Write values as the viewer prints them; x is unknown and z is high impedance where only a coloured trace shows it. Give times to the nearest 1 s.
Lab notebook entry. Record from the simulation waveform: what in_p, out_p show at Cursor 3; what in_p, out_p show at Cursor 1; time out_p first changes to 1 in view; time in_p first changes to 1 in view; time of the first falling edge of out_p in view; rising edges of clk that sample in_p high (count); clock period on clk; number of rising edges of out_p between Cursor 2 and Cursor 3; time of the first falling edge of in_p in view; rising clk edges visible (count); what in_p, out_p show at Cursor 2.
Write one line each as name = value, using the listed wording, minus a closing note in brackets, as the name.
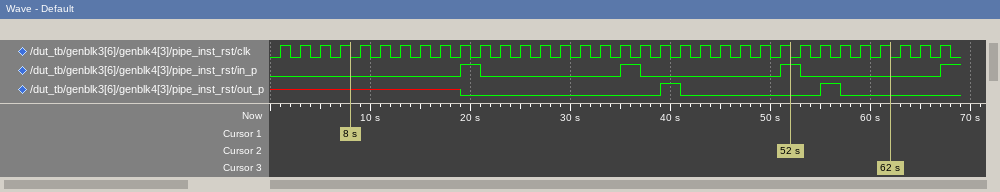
what in_p, out_p show at Cursor 3 = in_p=0, out_p=0
what in_p, out_p show at Cursor 1 = in_p=0, out_p=x
time out_p first changes to 1 in view = 39 s
time in_p first changes to 1 in view = 19 s
time of the first falling edge of out_p in view = 41 s
rising edges of clk that sample in_p high = 3
clock period on clk = 2 s
number of rising edges of out_p between Cursor 2 and Cursor 3 = 1
time of the first falling edge of in_p in view = 21 s
rising clk edges visible = 34
what in_p, out_p show at Cursor 2 = in_p=1, out_p=0
